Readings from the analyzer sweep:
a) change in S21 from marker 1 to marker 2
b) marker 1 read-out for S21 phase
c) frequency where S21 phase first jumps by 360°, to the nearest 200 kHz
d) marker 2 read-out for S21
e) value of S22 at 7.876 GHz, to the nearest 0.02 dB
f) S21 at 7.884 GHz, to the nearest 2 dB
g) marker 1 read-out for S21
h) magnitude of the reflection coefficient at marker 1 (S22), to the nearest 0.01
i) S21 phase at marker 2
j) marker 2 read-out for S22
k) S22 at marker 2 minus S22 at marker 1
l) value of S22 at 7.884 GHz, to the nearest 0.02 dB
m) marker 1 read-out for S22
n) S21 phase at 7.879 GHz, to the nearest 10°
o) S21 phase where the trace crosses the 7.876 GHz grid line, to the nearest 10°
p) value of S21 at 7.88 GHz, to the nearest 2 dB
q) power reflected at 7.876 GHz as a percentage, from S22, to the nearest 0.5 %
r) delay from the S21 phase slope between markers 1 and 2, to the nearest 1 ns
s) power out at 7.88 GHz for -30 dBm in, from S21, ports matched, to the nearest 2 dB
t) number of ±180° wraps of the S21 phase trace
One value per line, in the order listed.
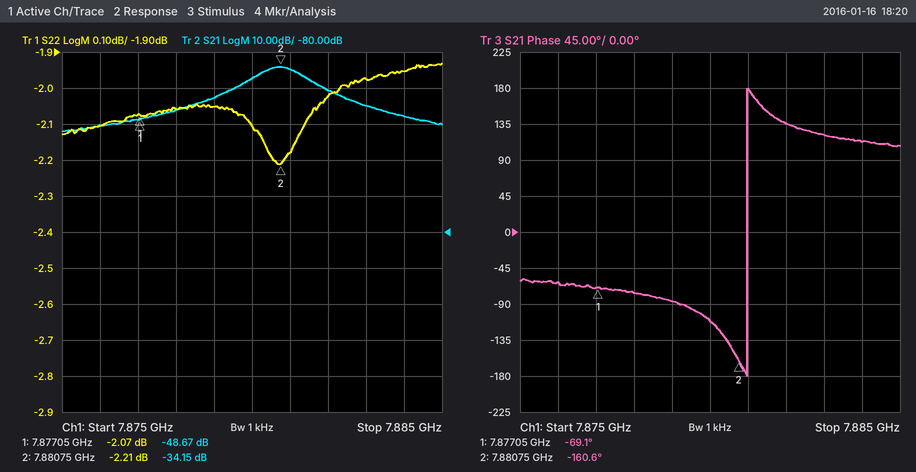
14.52 dB
-69.1°
7.8810 GHz
-34.15 dB
-2.10 dB
-48 dB
-48.67 dB
0.79
-160.6°
-2.21 dB
-0.14 dB
-1.96 dB
-2.07 dB
-90°
-60°
-38 dB
61.5 %
69 ns
-68 dBm
1
